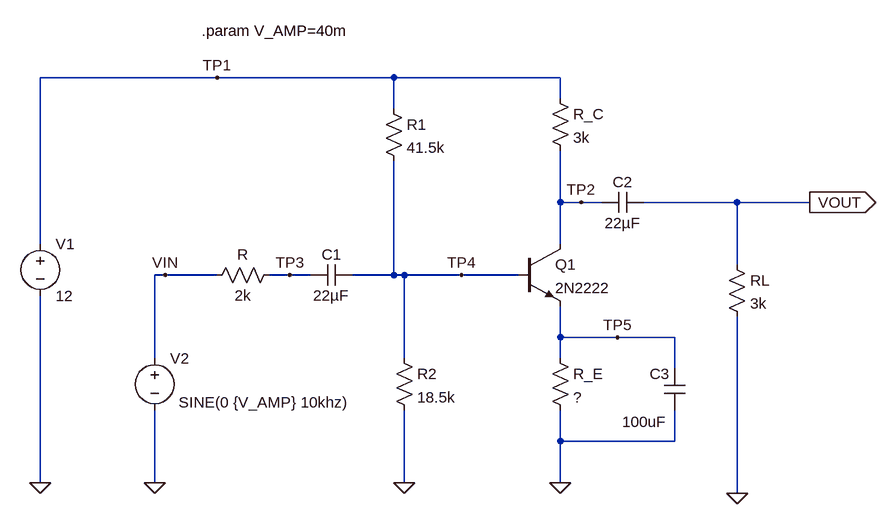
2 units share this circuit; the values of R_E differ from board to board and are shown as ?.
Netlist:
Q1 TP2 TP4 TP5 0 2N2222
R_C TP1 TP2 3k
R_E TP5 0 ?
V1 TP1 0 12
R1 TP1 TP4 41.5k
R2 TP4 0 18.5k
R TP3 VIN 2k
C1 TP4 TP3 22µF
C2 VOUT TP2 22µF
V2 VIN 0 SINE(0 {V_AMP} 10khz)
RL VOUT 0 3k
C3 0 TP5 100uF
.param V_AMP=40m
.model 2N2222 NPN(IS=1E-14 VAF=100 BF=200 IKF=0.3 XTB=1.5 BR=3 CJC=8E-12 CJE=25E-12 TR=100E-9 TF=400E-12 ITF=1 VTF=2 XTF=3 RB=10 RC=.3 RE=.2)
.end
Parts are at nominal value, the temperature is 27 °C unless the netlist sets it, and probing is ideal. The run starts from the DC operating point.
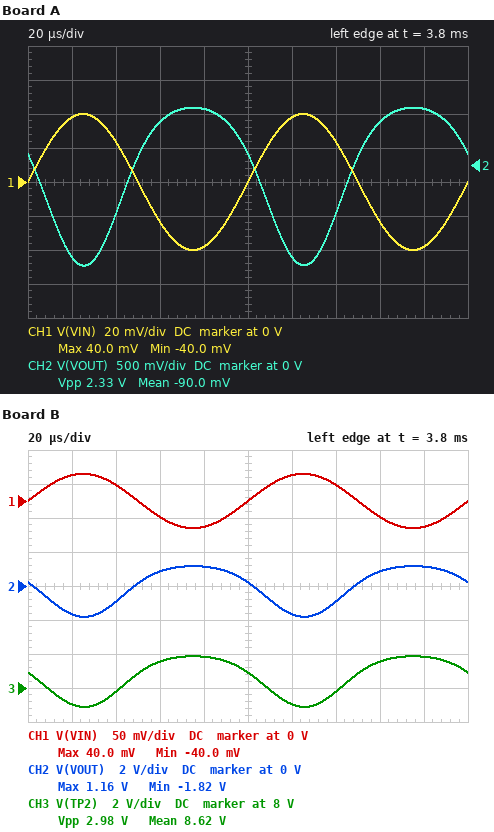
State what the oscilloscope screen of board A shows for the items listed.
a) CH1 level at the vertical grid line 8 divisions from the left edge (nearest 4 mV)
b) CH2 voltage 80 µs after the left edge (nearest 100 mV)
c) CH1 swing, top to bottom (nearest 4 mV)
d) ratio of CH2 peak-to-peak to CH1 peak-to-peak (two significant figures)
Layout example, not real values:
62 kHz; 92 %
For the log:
-24 mV; 800 mV; 80 mV; 29
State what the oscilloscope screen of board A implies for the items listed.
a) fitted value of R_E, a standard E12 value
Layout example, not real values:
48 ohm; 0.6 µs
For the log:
3.9 kΩ
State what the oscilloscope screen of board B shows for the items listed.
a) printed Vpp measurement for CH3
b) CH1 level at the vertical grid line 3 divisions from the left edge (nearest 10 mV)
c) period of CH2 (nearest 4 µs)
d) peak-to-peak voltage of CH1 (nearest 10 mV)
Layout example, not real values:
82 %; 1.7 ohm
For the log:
2.98 V; -20 mV; 100 µs; 80 mV
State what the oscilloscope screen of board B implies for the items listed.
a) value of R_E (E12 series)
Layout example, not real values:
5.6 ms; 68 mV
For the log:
2.7 kΩ
